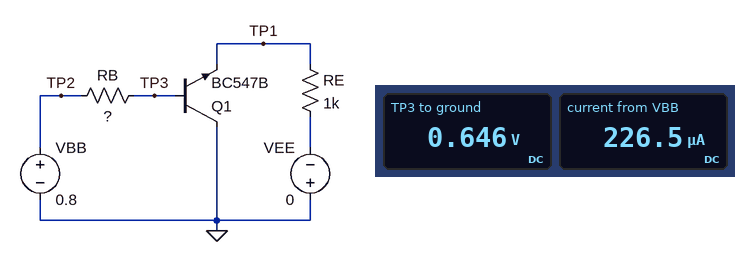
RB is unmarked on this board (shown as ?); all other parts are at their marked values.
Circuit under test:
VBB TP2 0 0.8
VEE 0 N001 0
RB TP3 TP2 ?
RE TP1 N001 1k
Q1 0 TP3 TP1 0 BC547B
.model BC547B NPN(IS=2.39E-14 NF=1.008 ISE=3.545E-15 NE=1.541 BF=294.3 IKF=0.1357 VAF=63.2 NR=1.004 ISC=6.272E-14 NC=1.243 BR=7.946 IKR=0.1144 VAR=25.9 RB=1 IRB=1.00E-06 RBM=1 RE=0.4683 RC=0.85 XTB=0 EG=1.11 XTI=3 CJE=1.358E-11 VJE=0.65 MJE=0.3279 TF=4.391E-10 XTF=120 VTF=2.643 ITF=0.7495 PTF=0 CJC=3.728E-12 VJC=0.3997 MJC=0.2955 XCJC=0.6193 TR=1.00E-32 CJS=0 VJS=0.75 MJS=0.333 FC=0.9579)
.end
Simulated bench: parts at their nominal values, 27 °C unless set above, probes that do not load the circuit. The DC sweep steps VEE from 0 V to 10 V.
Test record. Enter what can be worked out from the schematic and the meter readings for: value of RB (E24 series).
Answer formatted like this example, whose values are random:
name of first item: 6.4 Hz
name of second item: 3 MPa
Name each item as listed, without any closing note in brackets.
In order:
value of RB: 680 Ω
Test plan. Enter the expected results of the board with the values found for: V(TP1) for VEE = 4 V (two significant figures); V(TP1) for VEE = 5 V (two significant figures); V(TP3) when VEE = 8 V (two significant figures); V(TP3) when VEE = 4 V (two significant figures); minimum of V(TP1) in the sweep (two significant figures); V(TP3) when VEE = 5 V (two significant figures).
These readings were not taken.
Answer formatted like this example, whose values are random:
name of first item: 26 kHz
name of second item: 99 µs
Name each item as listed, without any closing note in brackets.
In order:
V(TP1) for VEE = 4 V: -44 mV
V(TP1) for VEE = 5 V: -50 mV
V(TP3) when VEE = 8 V: 640 mV
V(TP3) when VEE = 4 V: 640 mV
minimum of V(TP1) in the sweep: -74 mV
V(TP3) when VEE = 5 V: 640 mV
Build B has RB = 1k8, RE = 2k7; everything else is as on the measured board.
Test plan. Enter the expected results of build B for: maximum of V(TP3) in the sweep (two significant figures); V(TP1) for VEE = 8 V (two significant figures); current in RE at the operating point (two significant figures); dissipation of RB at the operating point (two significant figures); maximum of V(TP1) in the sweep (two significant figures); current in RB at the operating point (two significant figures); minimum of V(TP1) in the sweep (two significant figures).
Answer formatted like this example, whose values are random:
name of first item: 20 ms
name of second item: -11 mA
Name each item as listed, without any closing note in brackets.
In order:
maximum of V(TP3) in the sweep: 620 mV
V(TP1) for VEE = 8 V: -55 mV
current in RE at the operating point: 840 nA
dissipation of RB at the operating point: 17 µW
maximum of V(TP1) in the sweep: -2.3 mV
current in RB at the operating point: 98 µA
minimum of V(TP1) in the sweep: -61 mV
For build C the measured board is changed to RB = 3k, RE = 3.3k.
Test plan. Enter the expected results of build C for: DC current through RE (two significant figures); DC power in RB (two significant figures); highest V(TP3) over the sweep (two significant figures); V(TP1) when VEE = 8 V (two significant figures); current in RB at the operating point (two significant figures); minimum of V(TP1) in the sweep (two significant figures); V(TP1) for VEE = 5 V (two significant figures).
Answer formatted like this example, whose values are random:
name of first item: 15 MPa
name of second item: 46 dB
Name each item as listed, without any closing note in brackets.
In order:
DC current through RE: 680 nA
DC power in RB: 12 µW
highest V(TP3) over the sweep: 610 mV
V(TP1) when VEE = 8 V: -60 mV
current in RB at the operating point: 63 µA
minimum of V(TP1) in the sweep: -67 mV
V(TP1) for VEE = 5 V: -48 mV
